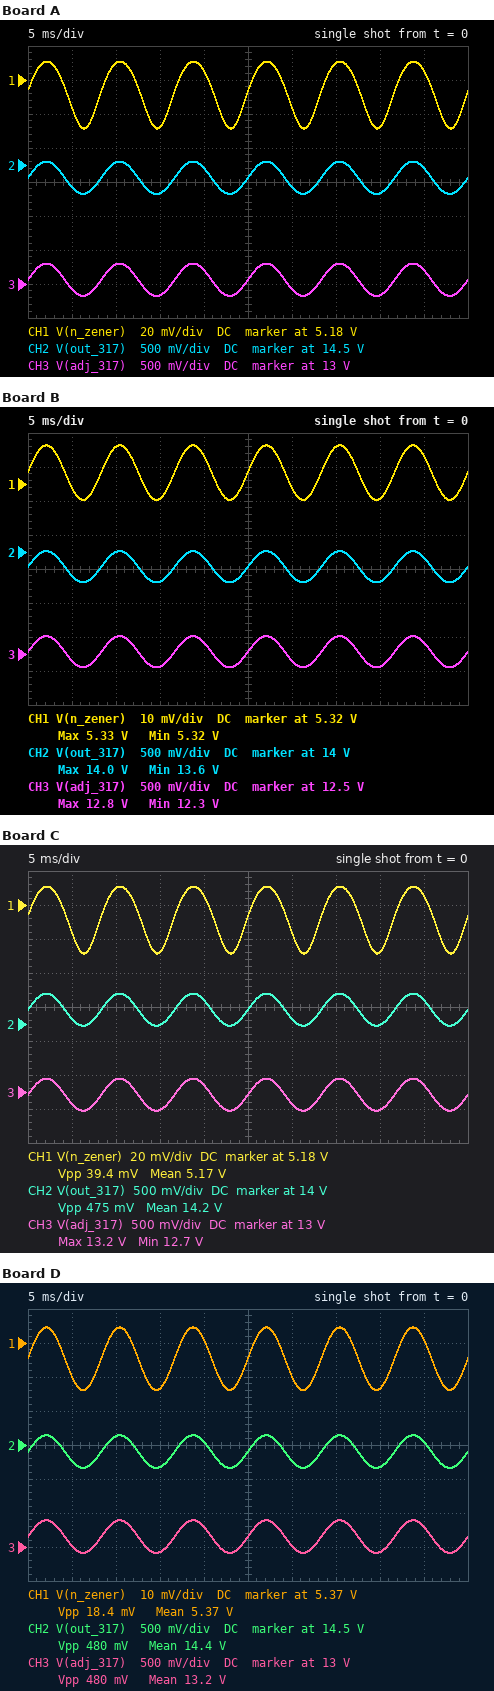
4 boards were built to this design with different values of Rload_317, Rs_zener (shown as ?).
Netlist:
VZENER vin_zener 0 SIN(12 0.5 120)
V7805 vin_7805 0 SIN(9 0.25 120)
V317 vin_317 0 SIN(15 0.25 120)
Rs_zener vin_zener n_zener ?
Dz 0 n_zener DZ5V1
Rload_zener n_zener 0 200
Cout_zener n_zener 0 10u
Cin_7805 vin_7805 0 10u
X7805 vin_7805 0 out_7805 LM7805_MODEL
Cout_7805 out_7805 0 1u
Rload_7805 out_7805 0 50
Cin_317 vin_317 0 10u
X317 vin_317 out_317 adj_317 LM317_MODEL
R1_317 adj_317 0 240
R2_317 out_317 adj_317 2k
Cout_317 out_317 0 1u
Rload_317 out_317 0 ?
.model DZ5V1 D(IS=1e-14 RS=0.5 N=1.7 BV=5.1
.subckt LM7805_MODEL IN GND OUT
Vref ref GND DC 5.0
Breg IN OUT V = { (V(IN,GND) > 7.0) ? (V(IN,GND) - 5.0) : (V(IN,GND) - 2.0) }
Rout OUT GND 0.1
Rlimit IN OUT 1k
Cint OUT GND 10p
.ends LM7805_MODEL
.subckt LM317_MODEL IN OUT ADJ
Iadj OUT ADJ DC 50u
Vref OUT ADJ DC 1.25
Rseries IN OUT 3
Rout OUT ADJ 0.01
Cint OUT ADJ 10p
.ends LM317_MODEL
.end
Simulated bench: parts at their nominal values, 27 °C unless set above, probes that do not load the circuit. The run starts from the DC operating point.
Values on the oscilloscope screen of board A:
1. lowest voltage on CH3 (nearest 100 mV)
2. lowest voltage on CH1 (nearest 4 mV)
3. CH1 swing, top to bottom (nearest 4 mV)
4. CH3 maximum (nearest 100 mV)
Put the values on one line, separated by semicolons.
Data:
12.8 V; 5.152 V; 40 mV; 13.3 V
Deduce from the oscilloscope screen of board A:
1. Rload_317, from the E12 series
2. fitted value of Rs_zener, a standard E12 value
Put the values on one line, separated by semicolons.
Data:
82 Ω; 220 Ω
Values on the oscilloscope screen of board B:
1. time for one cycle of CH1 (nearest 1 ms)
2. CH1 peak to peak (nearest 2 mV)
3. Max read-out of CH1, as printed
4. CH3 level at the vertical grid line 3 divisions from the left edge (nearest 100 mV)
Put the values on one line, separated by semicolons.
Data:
8 ms; 16 mV; 5.33 V; 12.3 V
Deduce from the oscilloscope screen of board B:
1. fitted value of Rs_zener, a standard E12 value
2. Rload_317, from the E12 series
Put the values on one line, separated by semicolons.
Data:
68 Ω; 39 Ω
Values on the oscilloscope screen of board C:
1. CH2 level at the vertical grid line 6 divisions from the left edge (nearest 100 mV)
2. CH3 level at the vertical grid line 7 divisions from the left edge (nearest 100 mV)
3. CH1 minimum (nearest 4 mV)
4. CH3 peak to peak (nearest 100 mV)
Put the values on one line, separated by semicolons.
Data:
14.1 V; 13.2 V; 5.152 V; 500 mV
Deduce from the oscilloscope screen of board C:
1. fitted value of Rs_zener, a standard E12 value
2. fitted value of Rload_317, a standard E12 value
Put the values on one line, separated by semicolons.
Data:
220 Ω; 68 Ω
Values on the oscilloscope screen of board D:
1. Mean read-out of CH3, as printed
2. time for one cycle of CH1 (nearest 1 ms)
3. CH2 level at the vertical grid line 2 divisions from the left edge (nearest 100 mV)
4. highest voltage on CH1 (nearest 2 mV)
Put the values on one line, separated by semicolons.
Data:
13.2 V; 8 ms; 14.6 V; 5.374 V
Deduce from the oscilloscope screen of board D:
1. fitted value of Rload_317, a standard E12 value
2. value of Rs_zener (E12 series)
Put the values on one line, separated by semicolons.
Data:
100 Ω; 47 Ω
